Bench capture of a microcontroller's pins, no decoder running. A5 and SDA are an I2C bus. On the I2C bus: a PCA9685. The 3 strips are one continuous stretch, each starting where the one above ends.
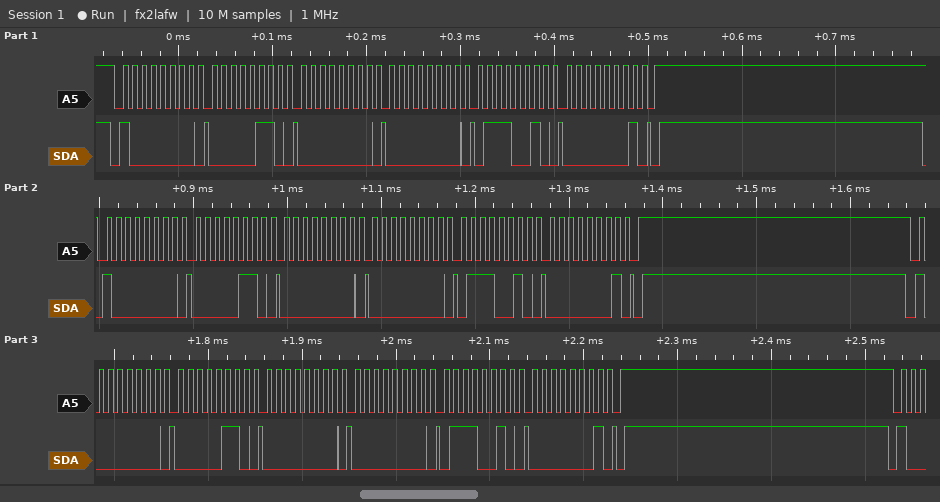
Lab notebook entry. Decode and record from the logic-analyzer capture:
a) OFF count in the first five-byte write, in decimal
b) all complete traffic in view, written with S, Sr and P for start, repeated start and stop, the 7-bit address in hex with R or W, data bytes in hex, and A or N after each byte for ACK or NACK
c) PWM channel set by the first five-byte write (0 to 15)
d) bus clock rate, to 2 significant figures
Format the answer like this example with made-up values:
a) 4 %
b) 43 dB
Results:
a) 370
b) S 40W A 06 A 00 A 00 A 72 A 01 A P S 40W A 06 A 00 A 00 A 72 A 01 A P S 40W A 06 A 00 A 00 A 72 A 01 A P
c) 0
d) 100 kHz
